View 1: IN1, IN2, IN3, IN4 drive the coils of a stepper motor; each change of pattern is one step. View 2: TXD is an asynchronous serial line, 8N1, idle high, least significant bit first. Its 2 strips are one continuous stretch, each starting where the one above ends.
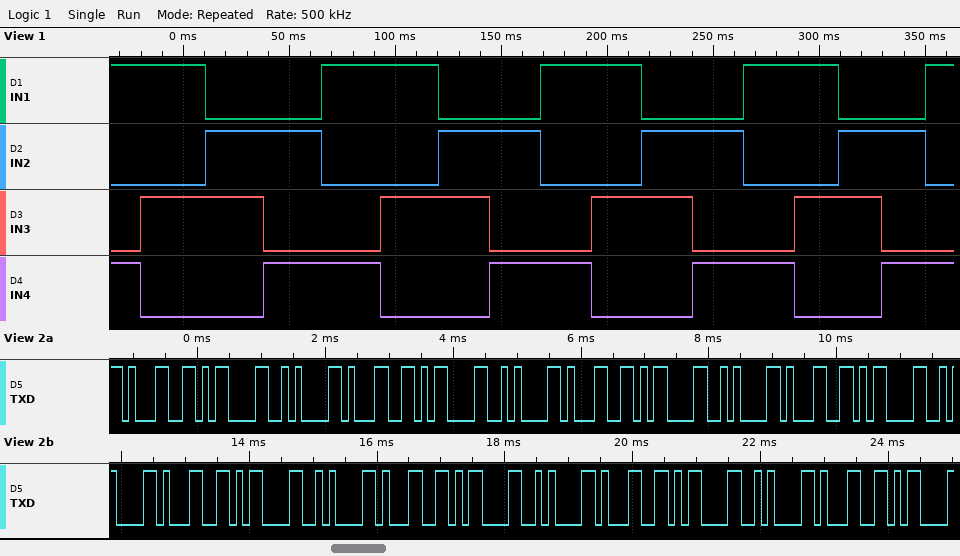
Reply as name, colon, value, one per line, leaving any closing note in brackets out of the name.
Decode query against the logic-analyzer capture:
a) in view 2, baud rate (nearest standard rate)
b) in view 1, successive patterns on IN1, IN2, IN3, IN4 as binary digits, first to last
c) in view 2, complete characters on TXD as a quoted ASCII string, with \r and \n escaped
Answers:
in view 2, baud rate: 9600 baud
in view 1, successive patterns on IN1, IN2, IN3, IN4 as binary digits, first to last: 1001 1010 0110 0101 1001 1010 0110 0101 1001 1010 0110 0101 1001 1010 0110 0101 1001
in view 2, complete characters on TXD as a quoted ASCII string, with \r and \n escaped: "1\r\n1\r\n1\r\n1\r\n1\r\n1\r\n1\r\n1\r"
